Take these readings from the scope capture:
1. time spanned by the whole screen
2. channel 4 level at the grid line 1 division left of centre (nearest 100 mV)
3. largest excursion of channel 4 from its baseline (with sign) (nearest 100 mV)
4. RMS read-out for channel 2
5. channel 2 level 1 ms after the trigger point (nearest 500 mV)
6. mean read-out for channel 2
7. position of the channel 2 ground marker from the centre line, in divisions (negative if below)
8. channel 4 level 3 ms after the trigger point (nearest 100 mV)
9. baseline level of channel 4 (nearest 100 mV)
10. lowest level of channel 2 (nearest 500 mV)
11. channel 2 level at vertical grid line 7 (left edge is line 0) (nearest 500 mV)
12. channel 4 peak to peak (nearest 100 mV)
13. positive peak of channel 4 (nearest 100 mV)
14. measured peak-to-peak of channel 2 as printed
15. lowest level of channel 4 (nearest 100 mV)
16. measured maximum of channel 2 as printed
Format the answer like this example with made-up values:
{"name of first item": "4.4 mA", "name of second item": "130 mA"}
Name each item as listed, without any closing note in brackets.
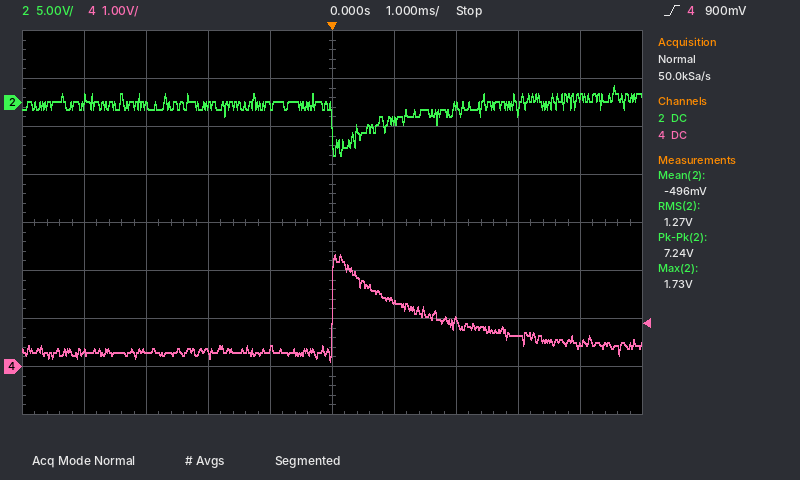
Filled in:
{"time spanned by the whole screen": "10 ms", "channel 4 level at the grid line 1 division left of centre": "400 mV", "largest excursion of channel 4 from its baseline (with sign)": "+2.0 V", "RMS read-out for channel 2": "1.27 V", "channel 2 level 1 ms after the trigger point": "-2.0 V", "mean read-out for channel 2": "-496 mV", "position of the channel 2 ground marker from the centre line, in divisions": "+2.5 div", "channel 4 level 3 ms after the trigger point": "600 mV", "baseline level of channel 4": "300 mV", "lowest level of channel 2": "-5.5 V", "channel 2 level at vertical grid line 7 (left edge is line 0)": "-500 mV", "channel 4 peak to peak": "2.2 V", "positive peak of channel 4": "2.3 V", "measured peak-to-peak of channel 2 as printed": "7.24 V", "lowest level of channel 4": "100 mV", "measured maximum of channel 2 as printed": "1.73 V"}
